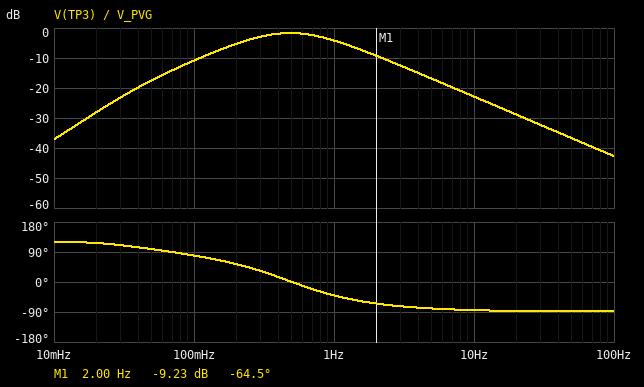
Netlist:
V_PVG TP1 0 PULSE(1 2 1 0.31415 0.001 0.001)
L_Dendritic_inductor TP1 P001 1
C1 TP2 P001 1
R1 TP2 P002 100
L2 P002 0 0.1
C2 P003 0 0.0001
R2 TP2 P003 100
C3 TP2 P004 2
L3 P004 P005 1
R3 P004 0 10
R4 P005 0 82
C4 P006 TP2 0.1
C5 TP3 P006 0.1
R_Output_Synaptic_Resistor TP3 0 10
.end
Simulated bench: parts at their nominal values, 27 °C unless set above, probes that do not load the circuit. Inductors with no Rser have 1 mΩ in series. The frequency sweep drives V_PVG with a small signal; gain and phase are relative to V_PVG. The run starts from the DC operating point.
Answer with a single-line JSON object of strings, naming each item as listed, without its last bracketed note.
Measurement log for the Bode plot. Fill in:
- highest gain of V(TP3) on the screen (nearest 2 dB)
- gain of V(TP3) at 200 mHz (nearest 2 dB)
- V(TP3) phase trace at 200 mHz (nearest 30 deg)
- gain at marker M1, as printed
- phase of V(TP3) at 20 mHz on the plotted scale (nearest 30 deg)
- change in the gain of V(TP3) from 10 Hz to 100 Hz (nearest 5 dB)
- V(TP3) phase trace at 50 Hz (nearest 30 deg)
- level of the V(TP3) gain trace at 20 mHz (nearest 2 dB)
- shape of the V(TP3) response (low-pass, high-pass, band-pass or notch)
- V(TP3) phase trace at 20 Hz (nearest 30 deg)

{"highest gain of V(TP3) on the screen": "-2 dB", "gain of V(TP3) at 200 mHz": "-6 dB", "V(TP3) phase trace at 200 mHz": "60 deg", "gain at marker M1, as printed": "-9.23 dB", "phase of V(TP3) at 20 mHz on the plotted scale": "120 deg", "change in the gain of V(TP3) from 10 Hz to 100 Hz": "-20 dB", "V(TP3) phase trace at 50 Hz": "-90 deg", "level of the V(TP3) gain trace at 20 mHz": "-28 dB", "shape of the V(TP3) response": "band-pass", "V(TP3) phase trace at 20 Hz": "-90 deg"}
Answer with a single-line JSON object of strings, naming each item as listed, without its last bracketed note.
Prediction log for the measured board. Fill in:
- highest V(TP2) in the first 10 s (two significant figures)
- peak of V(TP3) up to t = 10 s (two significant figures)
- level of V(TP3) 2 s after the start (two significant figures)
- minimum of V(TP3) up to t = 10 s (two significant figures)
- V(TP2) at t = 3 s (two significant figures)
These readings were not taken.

{"highest V(TP2) in the first 10 s": "500 mV", "peak of V(TP3) up to t = 10 s": "400 mV", "level of V(TP3) 2 s after the start": "-110 mV", "minimum of V(TP3) up to t = 10 s": "-120 mV", "V(TP2) at t = 3 s": "-20 mV"}
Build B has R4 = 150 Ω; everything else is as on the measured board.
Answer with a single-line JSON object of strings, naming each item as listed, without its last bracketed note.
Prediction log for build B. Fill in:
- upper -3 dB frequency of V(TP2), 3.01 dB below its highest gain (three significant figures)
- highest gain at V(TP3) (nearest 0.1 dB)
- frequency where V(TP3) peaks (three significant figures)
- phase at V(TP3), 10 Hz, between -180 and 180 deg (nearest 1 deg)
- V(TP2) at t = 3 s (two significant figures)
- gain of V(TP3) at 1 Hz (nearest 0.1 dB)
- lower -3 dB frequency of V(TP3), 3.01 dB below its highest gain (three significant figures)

{"upper -3 dB frequency of V(TP2), 3.01 dB below its highest gain": "861 mHz", "highest gain at V(TP3)": "-1.6 dB", "frequency where V(TP3) peaks": "493 mHz", "phase at V(TP3), 10 Hz, between -180 and 180 deg": "-85 deg", "V(TP2) at t = 3 s": "-19 mV", "gain of V(TP3) at 1 Hz": "-4.0 dB", "lower -3 dB frequency of V(TP3), 3.01 dB below its highest gain": "221 mHz"}
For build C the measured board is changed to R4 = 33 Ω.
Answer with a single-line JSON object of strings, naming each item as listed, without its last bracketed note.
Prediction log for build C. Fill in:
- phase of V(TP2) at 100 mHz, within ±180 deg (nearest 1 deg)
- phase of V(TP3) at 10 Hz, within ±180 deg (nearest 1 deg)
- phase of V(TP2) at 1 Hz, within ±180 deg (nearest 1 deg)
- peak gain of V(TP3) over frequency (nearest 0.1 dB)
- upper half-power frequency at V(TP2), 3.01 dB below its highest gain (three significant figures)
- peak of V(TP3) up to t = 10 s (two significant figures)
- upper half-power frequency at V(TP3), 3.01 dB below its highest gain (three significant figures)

{"phase of V(TP2) at 100 mHz, within ±180 deg": "8 deg", "phase of V(TP3) at 10 Hz, within ±180 deg": "-83 deg", "phase of V(TP2) at 1 Hz, within ±180 deg": "-59 deg", "peak gain of V(TP3) over frequency": "-1.9 dB", "upper half-power frequency at V(TP2), 3.01 dB below its highest gain": "784 mHz", "peak of V(TP3) up to t = 10 s": "380 mV", "upper half-power frequency at V(TP3), 3.01 dB below its highest gain": "1.03 Hz"}
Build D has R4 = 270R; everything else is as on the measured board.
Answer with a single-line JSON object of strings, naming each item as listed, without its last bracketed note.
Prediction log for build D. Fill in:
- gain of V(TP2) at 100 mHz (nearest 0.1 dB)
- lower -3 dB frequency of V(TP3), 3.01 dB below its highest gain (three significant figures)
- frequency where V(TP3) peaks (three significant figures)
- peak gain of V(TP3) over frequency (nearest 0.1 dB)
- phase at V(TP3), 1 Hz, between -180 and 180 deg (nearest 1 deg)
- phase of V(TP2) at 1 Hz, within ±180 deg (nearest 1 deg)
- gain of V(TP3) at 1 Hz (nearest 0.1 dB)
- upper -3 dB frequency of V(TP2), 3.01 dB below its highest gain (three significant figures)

{"gain of V(TP2) at 100 mHz": "-0.4 dB", "lower -3 dB frequency of V(TP3), 3.01 dB below its highest gain": "222 mHz", "frequency where V(TP3) peaks": "497 mHz", "peak gain of V(TP3) over frequency": "-1.6 dB", "phase at V(TP3), 1 Hz, between -180 and 180 deg": "-39 deg", "phase of V(TP2) at 1 Hz, within ±180 deg": "-57 deg", "gain of V(TP3) at 1 Hz": "-3.9 dB", "upper -3 dB frequency of V(TP2), 3.01 dB below its highest gain": "871 mHz"}
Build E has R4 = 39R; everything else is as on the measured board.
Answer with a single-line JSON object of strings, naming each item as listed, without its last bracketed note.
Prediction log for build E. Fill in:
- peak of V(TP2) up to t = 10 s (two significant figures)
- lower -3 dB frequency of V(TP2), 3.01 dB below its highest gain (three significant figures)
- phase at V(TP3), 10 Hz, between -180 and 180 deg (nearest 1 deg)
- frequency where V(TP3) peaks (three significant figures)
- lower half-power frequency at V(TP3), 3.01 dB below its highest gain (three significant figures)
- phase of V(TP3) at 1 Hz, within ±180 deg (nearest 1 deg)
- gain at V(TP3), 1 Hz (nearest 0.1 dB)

{"peak of V(TP2) up to t = 10 s": "480 mV", "lower -3 dB frequency of V(TP2), 3.01 dB below its highest gain": "31.9 mHz", "phase at V(TP3), 10 Hz, between -180 and 180 deg": "-83 deg", "frequency where V(TP3) peaks": "470 mHz", "lower half-power frequency at V(TP3), 3.01 dB below its highest gain": "213 mHz", "phase of V(TP3) at 1 Hz, within ±180 deg": "-41 deg", "gain at V(TP3), 1 Hz": "-4.6 dB"}
